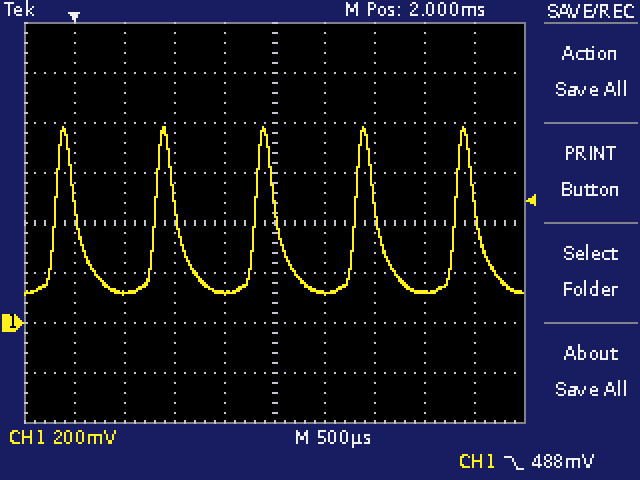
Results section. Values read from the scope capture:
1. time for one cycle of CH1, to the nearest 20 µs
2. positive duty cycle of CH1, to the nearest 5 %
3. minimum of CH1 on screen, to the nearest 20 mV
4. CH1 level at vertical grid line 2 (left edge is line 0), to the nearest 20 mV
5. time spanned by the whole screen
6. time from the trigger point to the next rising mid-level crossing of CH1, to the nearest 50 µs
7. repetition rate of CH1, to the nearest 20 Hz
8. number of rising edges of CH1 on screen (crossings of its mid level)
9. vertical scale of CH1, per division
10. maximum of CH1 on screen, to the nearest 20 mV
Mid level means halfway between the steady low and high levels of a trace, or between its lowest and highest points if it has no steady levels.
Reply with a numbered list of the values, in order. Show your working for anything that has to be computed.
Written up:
1. 1.00 ms
2. 20 %
3. 120 mV
4. 120 mV
5. 5 ms
6. 800 µs
7. 1 / 1.00 ms ≈ 1.00 kHz
8. 5
9. 200 mV
10. 780 mV
